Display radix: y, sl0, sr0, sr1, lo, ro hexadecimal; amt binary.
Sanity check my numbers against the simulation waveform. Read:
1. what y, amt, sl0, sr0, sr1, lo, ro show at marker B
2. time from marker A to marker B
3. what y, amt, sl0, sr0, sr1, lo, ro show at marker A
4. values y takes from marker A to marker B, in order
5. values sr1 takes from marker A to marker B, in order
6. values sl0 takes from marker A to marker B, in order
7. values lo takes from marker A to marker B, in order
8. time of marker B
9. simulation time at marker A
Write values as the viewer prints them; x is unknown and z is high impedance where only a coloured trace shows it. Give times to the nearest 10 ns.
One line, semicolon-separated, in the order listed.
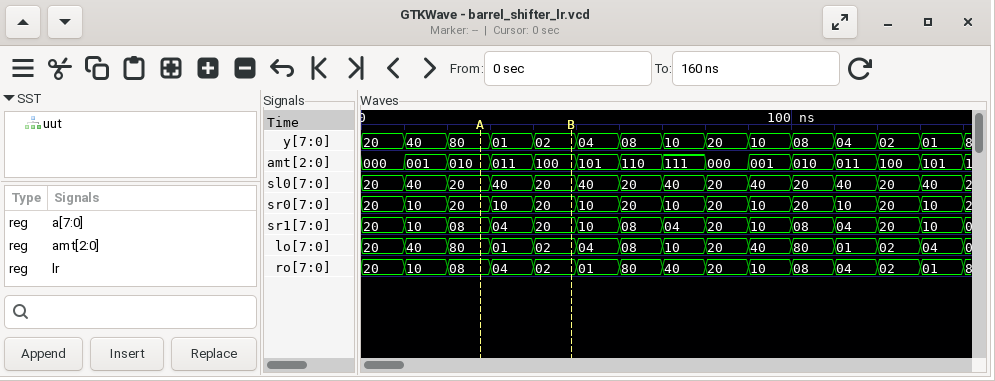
y=02, amt=100, sl0=20, sr0=20, sr1=20, lo=02, ro=02; 20 ns; y=80, amt=010, sl0=20, sr0=20, sr1=08, lo=80, ro=08; 80, 01, 02; 08, 04, 20; 20, 40, 20; 80, 01, 02; 50 ns; 30 ns
